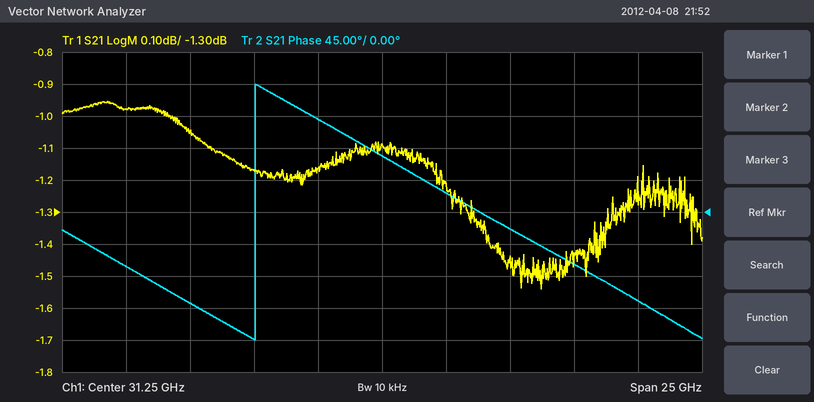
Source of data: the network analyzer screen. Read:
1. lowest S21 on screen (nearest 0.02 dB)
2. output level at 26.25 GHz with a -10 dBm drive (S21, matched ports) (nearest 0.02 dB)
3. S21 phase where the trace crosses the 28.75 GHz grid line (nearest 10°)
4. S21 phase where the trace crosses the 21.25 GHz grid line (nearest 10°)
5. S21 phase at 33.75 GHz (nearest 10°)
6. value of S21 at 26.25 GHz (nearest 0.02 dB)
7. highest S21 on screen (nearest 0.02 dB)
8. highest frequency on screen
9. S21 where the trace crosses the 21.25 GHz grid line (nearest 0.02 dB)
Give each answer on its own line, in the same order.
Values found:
-1.54 dB
-11.16 dBm
130°
-80°
30°
-1.16 dB
-0.96 dB
43.75 GHz
-0.98 dB
